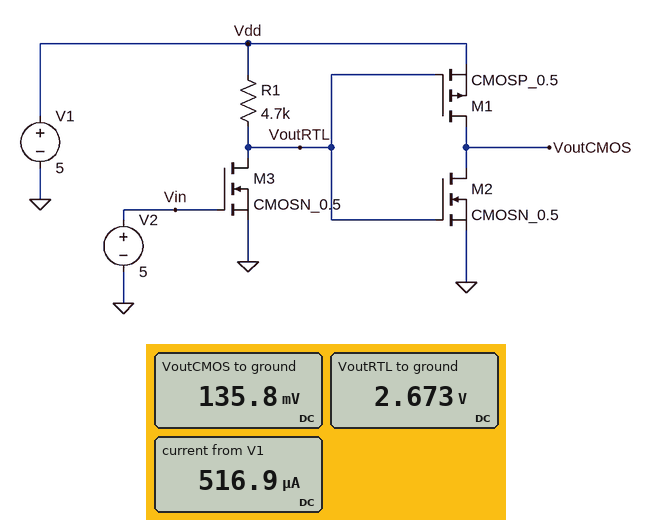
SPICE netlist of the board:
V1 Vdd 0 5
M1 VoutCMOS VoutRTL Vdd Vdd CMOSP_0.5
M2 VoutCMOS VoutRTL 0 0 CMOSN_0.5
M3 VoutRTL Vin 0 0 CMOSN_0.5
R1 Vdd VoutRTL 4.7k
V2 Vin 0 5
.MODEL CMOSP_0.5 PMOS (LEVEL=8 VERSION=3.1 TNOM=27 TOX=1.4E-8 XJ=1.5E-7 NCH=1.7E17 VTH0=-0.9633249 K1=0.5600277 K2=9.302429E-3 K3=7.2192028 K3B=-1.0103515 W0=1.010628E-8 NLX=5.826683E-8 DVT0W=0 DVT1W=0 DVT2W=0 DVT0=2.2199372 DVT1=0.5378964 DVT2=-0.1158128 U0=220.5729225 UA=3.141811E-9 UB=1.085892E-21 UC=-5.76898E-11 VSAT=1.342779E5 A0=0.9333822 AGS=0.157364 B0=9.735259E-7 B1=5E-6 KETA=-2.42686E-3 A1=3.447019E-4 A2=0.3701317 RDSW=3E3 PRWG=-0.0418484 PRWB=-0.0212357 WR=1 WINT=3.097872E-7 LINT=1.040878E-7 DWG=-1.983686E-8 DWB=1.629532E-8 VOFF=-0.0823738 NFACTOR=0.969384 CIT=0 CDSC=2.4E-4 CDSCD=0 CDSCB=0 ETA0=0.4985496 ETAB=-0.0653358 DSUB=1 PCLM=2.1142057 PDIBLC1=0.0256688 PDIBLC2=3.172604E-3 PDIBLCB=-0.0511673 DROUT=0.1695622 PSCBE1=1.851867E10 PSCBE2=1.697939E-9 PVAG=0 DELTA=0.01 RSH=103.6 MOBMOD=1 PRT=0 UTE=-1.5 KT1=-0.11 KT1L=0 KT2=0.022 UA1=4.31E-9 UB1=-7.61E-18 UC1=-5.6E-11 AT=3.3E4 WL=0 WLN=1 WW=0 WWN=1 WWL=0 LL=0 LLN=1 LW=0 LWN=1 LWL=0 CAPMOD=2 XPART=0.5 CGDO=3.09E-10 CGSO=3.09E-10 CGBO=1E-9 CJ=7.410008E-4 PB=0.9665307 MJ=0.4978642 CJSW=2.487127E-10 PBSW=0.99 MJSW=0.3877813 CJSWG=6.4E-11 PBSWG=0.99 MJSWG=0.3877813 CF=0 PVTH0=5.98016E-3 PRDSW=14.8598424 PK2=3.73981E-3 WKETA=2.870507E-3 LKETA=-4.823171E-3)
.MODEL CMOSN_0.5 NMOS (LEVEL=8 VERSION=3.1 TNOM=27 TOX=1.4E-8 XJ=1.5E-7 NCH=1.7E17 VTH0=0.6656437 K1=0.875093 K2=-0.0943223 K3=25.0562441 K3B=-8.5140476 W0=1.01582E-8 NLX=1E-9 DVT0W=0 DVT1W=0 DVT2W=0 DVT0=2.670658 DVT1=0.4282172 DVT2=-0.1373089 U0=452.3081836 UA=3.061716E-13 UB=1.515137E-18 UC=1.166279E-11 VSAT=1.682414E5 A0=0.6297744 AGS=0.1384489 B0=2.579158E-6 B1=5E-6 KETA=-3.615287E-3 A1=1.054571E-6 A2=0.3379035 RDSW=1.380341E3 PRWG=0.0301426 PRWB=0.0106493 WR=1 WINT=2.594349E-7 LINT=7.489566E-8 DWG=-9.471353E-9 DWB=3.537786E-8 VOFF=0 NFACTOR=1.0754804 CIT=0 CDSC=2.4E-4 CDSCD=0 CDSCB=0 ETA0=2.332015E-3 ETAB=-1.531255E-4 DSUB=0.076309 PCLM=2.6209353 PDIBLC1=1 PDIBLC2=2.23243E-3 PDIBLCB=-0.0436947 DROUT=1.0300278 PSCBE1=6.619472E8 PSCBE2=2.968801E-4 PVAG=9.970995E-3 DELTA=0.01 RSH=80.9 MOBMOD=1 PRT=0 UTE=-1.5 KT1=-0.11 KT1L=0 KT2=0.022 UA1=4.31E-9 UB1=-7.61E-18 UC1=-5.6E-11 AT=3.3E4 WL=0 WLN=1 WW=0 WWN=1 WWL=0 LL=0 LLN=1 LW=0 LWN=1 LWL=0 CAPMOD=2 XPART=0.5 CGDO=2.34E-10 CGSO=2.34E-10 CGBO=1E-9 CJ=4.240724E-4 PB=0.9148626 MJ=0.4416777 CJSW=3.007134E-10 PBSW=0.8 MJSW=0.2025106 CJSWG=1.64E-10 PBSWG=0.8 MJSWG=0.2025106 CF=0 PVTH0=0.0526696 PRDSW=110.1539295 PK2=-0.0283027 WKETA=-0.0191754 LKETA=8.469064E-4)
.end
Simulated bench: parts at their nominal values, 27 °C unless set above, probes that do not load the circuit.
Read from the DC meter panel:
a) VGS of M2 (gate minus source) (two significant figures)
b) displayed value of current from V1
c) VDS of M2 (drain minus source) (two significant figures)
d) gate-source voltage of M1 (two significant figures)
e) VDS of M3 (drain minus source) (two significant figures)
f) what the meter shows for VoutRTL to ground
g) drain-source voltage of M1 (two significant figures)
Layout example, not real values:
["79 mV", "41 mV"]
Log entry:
["2.7 V", "516.9 µA", "140 mV", "-2.3 V", "2.7 V", "2.673 V", "-4.9 V"]
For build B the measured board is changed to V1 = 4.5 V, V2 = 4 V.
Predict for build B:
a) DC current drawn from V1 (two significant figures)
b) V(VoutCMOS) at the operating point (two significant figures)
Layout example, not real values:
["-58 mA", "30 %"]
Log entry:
["330 µA", "24 mV"]
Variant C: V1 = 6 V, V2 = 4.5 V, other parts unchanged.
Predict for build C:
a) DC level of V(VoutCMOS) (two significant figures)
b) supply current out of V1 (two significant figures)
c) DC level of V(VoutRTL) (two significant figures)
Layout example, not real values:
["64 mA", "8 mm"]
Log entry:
["52 mV", "440 µA", "4.0 V"]
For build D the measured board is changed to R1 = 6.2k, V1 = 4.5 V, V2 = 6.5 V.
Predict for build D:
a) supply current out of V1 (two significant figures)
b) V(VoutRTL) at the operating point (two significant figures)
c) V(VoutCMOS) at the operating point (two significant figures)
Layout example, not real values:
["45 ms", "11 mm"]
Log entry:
["500 µA", "1.6 V", "3.8 V"]
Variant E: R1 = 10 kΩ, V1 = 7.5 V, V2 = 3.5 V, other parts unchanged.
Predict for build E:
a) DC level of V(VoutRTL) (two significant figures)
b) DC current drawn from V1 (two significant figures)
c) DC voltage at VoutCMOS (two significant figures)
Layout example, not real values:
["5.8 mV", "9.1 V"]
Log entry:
["5.0 V", "280 µA", "91 mV"]
